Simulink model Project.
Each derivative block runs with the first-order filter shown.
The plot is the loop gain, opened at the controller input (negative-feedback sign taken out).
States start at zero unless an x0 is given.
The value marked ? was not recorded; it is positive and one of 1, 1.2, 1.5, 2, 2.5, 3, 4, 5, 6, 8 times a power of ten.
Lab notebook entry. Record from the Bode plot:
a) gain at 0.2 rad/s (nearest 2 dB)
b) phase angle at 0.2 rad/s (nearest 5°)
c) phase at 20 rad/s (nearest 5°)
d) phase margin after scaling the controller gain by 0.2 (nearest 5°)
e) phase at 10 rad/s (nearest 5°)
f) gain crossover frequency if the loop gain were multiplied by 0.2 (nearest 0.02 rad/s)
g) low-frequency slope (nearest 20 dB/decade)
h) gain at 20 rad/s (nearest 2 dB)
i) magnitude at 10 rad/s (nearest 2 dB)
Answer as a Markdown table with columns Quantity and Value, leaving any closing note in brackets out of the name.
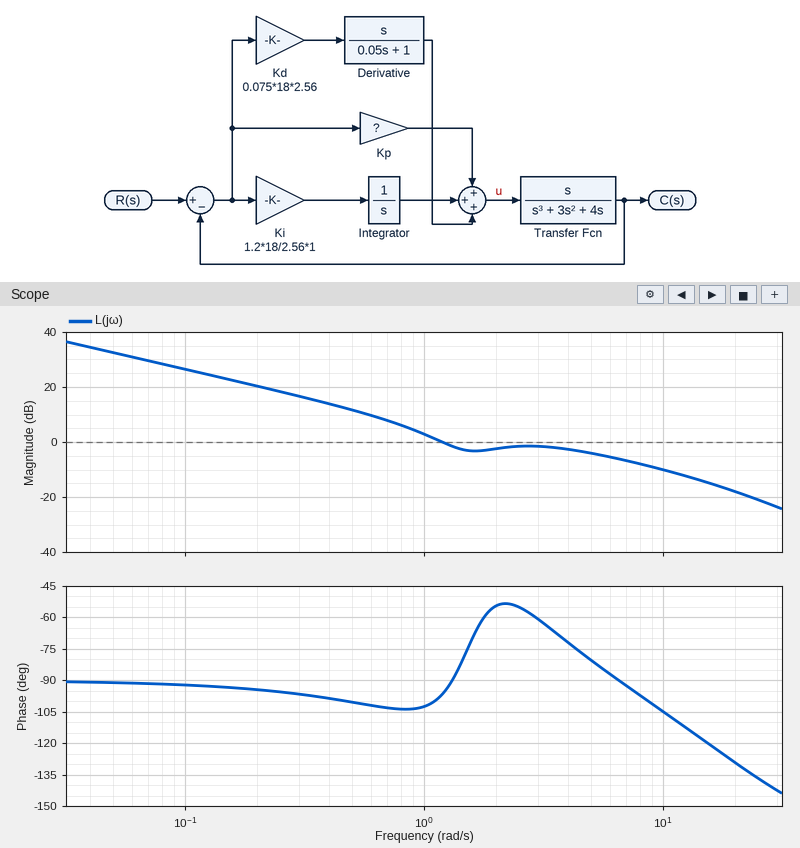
| Quantity | Value |
|---|---|
| gain at 0.2 rad/s | 20 dB |
| phase angle at 0.2 rad/s | -95° |
| phase at 20 rad/s | -130° |
| phase margin after scaling the controller gain by 0.2 | 80° |
| phase at 10 rad/s | -105° |
| gain crossover frequency if the loop gain were multiplied by 0.2 | 0.40 rad/s |
| low-frequency slope | -20 dB/decade |
| gain at 20 rad/s | -18 dB |
| magnitude at 10 rad/s | -10 dB |
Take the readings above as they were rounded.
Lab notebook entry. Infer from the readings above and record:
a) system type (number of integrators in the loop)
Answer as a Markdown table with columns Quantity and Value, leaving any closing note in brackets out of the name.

| Quantity | Value |
|---|---|
| system type | 1 |
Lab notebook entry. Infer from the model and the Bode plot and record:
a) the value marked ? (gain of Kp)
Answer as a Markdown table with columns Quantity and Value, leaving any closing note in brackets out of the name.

| Quantity | Value |
|---|---|
| the value marked ? | 3 |
